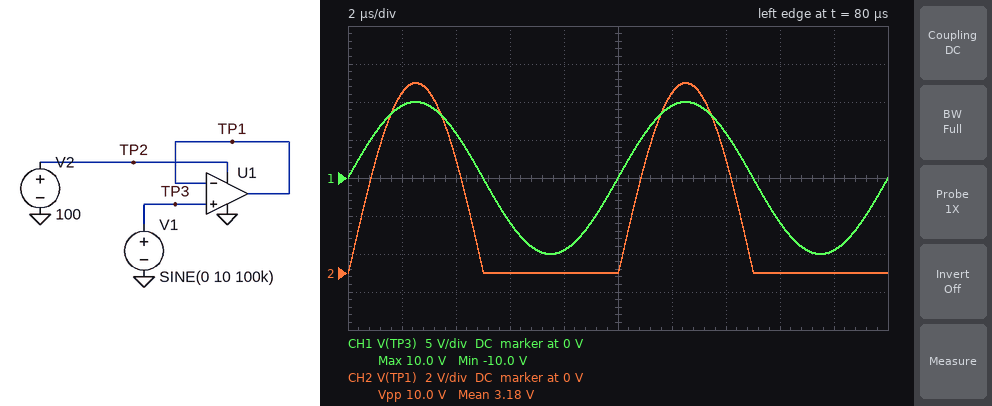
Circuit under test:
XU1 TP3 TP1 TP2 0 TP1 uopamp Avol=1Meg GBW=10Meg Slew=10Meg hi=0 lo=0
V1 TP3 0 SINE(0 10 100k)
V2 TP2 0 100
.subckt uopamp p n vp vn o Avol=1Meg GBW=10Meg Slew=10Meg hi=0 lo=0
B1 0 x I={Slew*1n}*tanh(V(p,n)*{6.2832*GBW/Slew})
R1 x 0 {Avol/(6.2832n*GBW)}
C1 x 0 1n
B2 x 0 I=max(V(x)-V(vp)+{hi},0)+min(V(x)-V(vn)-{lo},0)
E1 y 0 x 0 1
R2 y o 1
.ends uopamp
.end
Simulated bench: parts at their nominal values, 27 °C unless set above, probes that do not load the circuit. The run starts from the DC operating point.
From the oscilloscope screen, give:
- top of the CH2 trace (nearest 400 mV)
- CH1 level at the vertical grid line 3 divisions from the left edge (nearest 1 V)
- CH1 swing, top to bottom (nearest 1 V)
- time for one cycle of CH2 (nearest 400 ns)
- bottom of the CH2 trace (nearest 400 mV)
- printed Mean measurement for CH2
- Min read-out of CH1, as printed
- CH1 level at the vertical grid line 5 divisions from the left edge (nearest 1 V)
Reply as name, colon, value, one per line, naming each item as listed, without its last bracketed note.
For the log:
top of the CH2 trace: 10.0 V
CH1 level at the vertical grid line 3 divisions from the left edge: -6 V
CH1 swing, top to bottom: 20 V
time for one cycle of CH2: 10.0 µs
bottom of the CH2 trace: 0 V
printed Mean measurement for CH2: 3.18 V
Min read-out of CH1, as printed: -10.0 V
CH1 level at the vertical grid line 5 divisions from the left edge: 0 V
